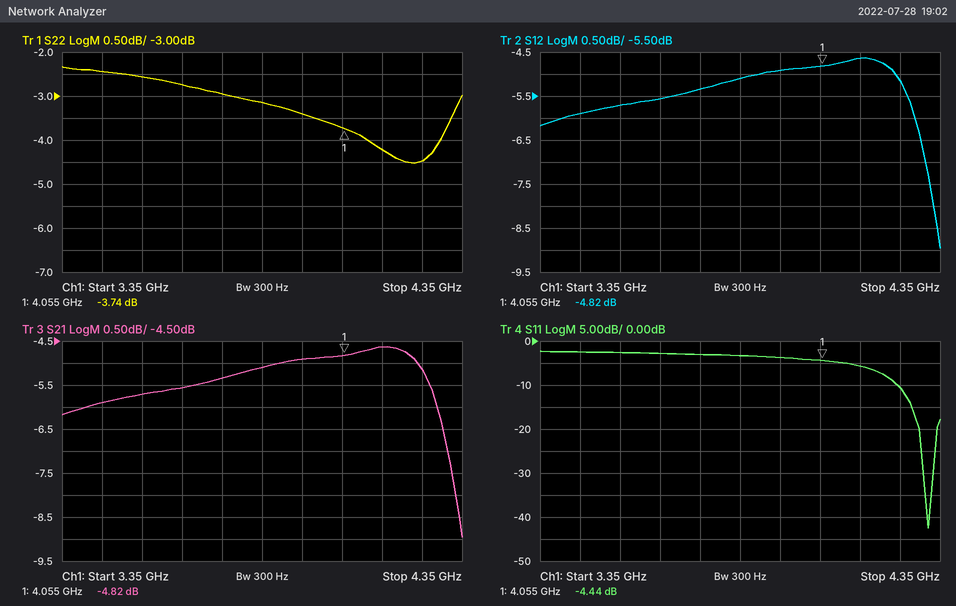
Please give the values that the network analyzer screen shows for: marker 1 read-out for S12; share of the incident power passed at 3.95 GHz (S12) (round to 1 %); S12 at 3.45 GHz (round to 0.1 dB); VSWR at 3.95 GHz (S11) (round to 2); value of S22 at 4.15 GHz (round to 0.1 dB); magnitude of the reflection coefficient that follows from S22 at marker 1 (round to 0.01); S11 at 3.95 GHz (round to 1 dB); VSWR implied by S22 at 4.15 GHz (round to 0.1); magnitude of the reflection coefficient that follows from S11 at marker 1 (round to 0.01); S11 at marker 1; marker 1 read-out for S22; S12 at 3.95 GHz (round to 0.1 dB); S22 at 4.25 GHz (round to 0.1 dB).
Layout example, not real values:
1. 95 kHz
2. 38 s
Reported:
1. -4.82 dB
2. 32 %
3. -5.9 dB
4. 4
5. -4.2 dB
6. 0.65
7. -4 dB
8. 4.2
9. 0.60
10. -4.44 dB
11. -3.74 dB
12. -4.9 dB
13. -4.5 dB
